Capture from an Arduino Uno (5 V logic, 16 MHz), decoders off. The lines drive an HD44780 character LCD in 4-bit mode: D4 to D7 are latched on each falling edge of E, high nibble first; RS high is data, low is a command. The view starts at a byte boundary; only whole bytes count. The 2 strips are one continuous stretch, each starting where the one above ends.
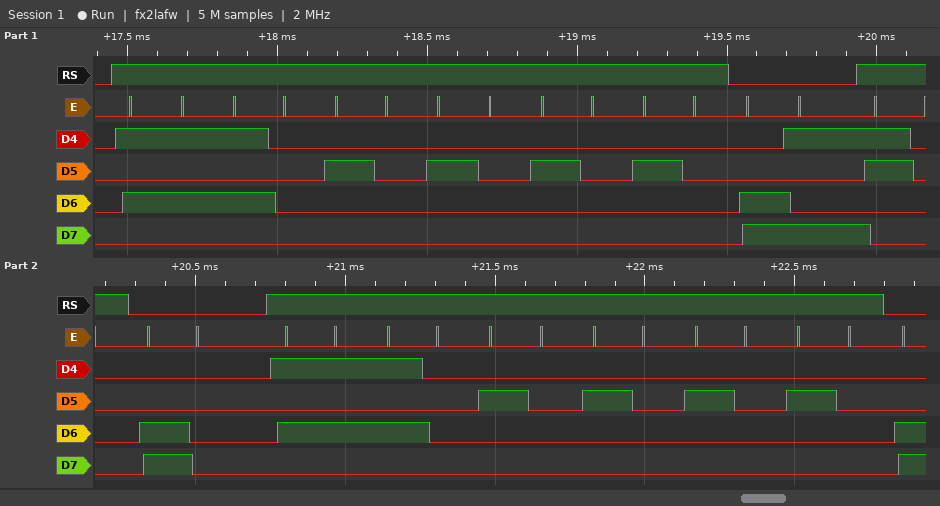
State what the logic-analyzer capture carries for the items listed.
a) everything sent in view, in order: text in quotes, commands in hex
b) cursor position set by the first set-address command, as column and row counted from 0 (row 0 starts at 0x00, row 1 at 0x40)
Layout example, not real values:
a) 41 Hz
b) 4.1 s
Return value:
a) "UP    " 0xC9 "0" 0xC0 "UP    "
b) column 9, row 1
